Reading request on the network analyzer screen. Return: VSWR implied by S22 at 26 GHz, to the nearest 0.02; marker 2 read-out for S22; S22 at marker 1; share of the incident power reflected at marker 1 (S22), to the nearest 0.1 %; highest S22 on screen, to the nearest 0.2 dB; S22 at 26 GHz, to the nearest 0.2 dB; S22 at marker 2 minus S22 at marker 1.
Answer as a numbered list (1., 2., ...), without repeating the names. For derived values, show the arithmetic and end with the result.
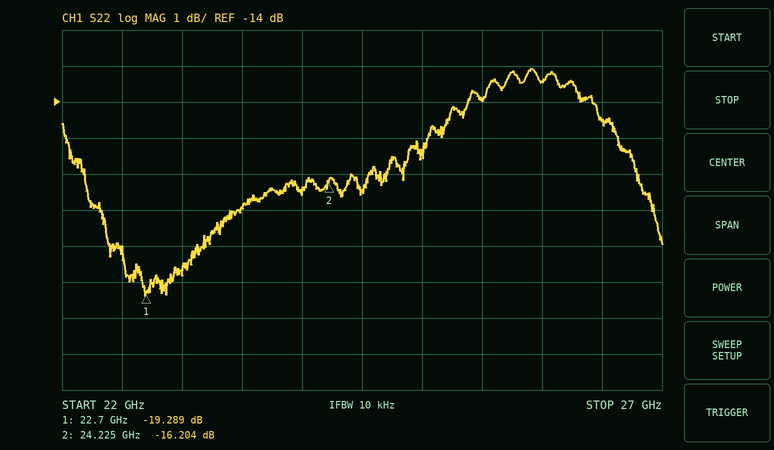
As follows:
1. |Γ| = 10^(-13.4/20) = 0.2138; VSWR = (1 + 0.2138)/(1 − 0.2138) ≈ 1.54
2. -16.204 dB
3. -19.289 dB
4. 10^(-19.289/10) ≈ 1.2 %
5. -13.0 dB
6. -13.4 dB
7. -16.204 − (-19.289) = 3.085 dB
